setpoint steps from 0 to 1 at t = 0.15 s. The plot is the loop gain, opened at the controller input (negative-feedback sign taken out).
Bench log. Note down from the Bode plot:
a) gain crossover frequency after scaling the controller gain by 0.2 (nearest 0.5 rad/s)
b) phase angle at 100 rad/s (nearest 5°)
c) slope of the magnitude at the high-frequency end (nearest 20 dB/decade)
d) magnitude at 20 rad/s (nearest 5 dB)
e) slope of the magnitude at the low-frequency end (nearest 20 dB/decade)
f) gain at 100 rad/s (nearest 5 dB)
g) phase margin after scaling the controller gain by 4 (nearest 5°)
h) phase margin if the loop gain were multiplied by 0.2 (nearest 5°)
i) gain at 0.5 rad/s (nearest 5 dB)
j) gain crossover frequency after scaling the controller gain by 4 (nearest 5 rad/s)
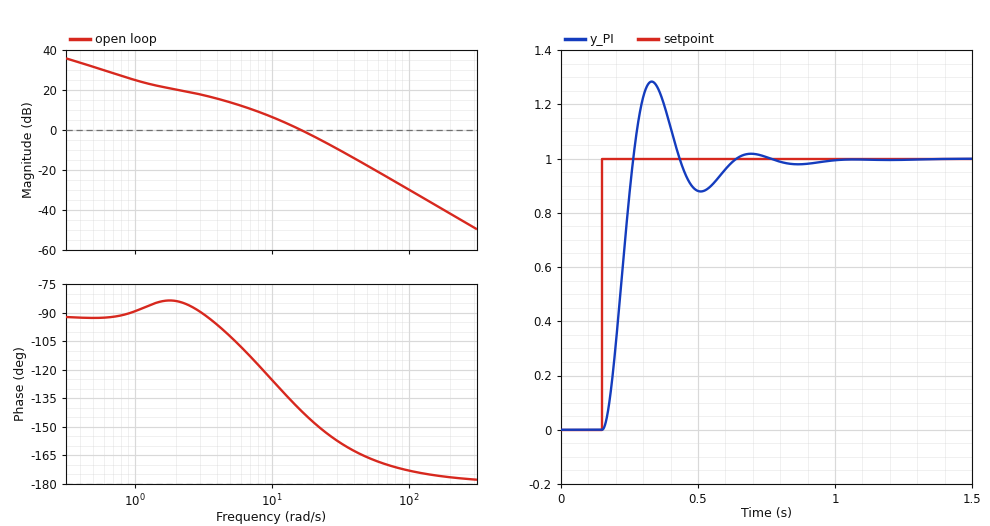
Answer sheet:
5.0 rad/s
-175°
-40 dB/decade
-5 dB
-20 dB/decade
-30 dB
20°
80°
30 dB
35 rad/s
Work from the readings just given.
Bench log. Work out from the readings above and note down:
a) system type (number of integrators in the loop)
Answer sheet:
1
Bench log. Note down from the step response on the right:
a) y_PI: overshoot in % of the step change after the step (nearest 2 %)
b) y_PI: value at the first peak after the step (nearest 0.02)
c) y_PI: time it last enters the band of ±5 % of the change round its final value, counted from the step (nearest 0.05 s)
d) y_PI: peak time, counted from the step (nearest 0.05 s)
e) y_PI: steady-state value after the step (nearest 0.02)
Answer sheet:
28 %
1.28
0.45 s
0.20 s
1.00
